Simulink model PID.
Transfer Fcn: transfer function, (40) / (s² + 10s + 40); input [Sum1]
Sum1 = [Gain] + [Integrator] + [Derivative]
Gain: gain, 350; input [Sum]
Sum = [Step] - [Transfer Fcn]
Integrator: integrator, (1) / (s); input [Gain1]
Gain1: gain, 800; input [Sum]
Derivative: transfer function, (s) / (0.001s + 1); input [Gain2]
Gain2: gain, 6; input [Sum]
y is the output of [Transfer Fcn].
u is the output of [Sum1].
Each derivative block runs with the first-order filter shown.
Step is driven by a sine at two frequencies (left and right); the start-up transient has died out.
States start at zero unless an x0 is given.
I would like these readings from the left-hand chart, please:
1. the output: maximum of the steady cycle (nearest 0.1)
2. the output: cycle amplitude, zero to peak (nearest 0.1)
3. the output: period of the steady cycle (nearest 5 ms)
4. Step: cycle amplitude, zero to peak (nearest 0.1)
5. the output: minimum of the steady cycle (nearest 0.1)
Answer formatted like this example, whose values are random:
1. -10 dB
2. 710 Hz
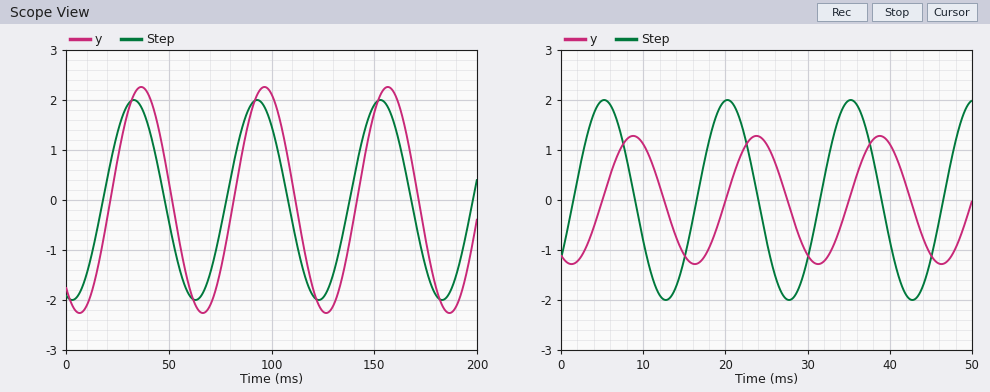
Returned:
1. 2.3
2. 2.3
3. 60 ms
4. 2.0
5. -2.3
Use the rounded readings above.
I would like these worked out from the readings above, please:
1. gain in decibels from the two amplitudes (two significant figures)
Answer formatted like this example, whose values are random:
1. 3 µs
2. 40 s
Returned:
1. 1.2 dB
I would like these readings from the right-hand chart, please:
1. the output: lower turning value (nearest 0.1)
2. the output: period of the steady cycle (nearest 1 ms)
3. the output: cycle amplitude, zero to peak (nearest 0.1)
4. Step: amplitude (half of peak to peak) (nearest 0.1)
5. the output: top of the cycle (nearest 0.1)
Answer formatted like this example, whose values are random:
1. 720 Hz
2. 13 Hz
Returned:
1. -1.3
2. 15 ms
3. 1.3
4. 2.0
5. 1.3
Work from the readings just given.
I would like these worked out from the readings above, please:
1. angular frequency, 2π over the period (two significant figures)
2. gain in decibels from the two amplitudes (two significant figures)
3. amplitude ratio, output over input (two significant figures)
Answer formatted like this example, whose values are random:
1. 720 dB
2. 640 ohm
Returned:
1. 0.42 rad/ms
2. -3.7 dB
3. 0.65
